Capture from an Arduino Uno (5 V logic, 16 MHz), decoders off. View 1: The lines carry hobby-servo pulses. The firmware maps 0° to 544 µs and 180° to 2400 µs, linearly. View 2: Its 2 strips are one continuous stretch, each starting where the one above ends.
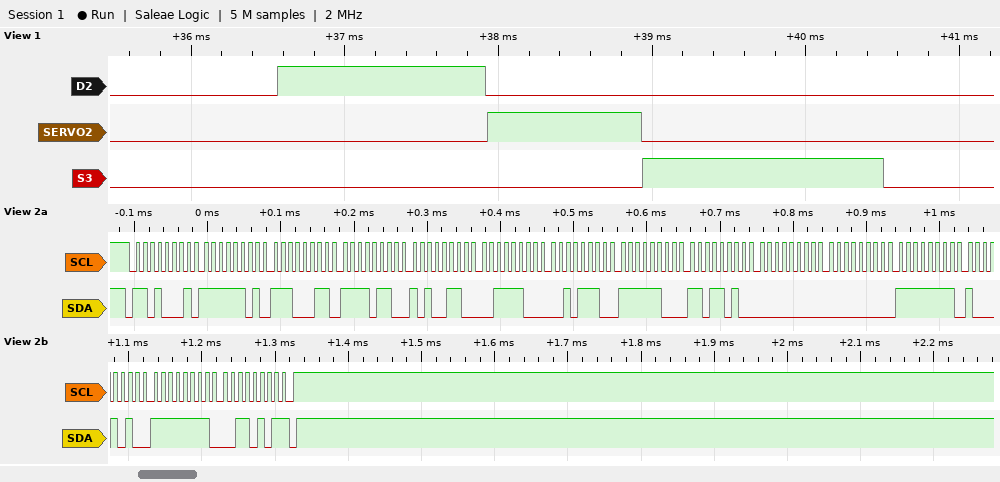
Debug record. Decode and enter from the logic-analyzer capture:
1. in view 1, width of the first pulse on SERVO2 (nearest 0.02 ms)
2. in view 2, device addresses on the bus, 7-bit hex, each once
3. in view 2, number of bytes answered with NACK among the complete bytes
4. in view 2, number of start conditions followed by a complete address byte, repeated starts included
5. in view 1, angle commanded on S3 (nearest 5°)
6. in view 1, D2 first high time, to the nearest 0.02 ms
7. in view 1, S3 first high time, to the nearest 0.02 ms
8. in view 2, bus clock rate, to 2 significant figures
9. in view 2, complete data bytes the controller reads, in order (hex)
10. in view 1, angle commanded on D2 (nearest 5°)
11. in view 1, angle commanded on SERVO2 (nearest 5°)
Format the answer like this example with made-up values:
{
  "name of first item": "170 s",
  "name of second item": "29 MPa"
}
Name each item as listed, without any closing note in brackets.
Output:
{
  "in view 1, width of the first pulse on SERVO2": "1.00 ms",
  "in view 2, device addresses on the bus, 7-bit hex, each once": "0x68",
  "in view 2, number of bytes answered with NACK among the complete bytes": "1",
  "in view 2, number of start conditions followed by a complete address byte, repeated starts included": "1",
  "in view 1, angle commanded on S3": "100°",
  "in view 1, D2 first high time, to the nearest 0.02 ms": "1.36 ms",
  "in view 1, S3 first high time, to the nearest 0.02 ms": "1.56 ms",
  "in view 2, bus clock rate, to 2 significant figures": "100 kHz",
  "in view 2, complete data bytes the controller reads, in order": "FD E3 F6 A6 3C 2E FC DA 00 00 FF 8A FF 35",
  "in view 1, angle commanded on D2": "80°",
  "in view 1, angle commanded on SERVO2": "45°"
}
